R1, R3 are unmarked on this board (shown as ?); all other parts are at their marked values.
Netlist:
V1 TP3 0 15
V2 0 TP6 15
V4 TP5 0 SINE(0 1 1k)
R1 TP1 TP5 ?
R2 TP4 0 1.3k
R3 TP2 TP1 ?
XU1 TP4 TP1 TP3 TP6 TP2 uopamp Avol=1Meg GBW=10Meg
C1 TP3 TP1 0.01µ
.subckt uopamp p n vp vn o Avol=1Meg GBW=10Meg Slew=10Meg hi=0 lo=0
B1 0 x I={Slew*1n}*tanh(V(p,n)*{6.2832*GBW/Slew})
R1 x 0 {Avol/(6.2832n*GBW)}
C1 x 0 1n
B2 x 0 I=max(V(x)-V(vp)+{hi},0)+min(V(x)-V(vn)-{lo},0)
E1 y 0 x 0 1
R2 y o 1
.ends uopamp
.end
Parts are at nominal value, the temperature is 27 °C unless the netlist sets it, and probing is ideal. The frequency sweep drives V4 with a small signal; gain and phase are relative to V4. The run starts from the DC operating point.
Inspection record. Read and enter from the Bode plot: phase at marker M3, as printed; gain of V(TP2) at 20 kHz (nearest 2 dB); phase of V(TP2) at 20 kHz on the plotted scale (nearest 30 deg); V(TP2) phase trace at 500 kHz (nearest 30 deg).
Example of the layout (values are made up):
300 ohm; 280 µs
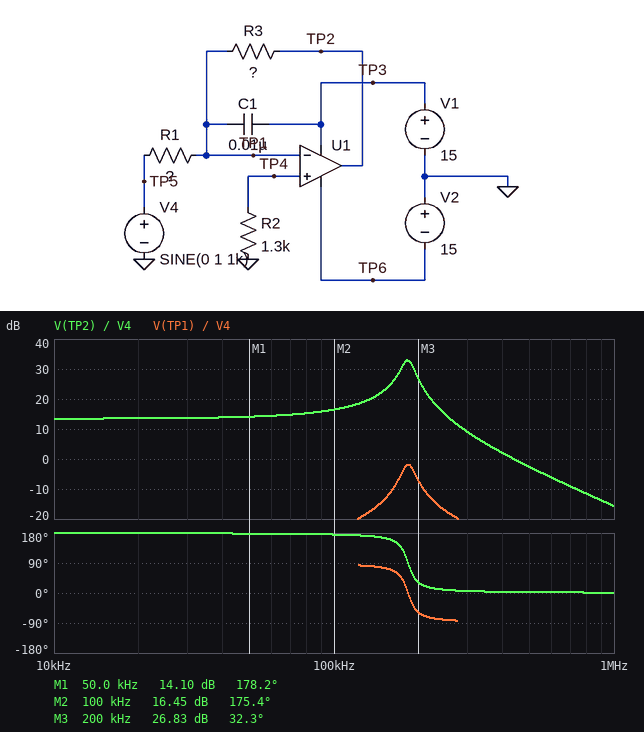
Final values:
32.3 deg; 14 dB; 180 deg; 0 deg
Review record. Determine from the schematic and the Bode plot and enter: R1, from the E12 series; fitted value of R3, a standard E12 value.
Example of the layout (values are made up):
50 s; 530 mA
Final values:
1 kΩ; 4.7 kΩ
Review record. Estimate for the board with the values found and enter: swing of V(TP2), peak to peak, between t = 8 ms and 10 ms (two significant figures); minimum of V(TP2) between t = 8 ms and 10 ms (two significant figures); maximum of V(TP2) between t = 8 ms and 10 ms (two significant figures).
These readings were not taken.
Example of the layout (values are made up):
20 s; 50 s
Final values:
9.4 V; -4.7 V; 4.7 V
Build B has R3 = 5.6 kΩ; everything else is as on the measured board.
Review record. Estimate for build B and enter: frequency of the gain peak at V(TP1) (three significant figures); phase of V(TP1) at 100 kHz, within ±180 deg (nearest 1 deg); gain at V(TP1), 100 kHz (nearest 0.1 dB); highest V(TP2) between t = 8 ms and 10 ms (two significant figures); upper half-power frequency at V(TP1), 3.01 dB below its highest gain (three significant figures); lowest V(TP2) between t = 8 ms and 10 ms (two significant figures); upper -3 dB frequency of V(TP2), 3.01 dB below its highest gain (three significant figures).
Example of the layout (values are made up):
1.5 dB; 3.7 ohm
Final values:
169 kHz; 84 deg; -21.3 dB; 5.6 V; 178 kHz; -5.6 V; 177 kHz
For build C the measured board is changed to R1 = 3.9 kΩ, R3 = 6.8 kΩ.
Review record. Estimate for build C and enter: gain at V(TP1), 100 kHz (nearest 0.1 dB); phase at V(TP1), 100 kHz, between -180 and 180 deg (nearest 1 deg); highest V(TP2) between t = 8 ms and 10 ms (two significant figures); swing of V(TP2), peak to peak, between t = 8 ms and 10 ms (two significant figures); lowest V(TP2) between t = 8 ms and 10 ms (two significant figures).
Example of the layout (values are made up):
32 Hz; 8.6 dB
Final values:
-30.3 dB; 87 deg; 1.7 V; 3.5 V; -1.7 V
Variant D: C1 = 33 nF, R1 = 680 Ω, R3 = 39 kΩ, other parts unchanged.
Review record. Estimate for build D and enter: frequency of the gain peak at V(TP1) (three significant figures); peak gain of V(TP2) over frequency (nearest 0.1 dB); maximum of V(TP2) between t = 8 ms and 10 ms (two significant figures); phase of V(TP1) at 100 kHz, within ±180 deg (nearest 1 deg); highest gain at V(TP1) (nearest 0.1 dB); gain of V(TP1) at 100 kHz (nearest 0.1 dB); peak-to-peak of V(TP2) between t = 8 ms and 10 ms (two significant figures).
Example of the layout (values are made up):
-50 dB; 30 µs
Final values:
35.2 kHz; 49.0 dB; 15 V; -85 deg; -0.2 dB; -21.9 dB; 30 V
